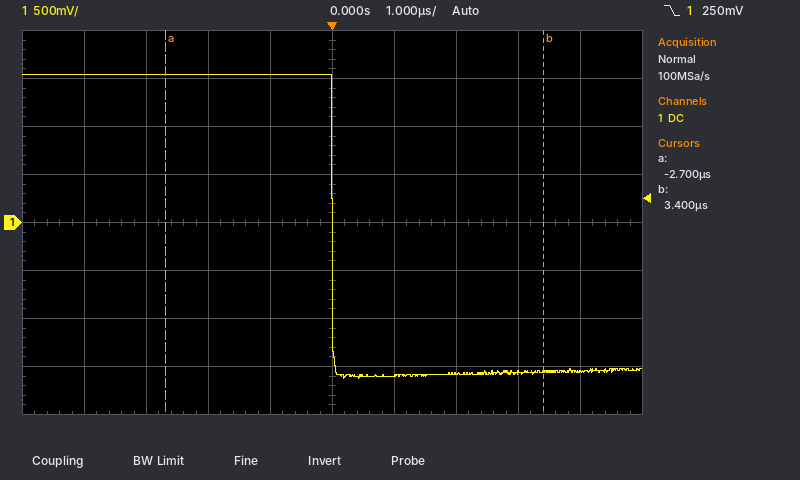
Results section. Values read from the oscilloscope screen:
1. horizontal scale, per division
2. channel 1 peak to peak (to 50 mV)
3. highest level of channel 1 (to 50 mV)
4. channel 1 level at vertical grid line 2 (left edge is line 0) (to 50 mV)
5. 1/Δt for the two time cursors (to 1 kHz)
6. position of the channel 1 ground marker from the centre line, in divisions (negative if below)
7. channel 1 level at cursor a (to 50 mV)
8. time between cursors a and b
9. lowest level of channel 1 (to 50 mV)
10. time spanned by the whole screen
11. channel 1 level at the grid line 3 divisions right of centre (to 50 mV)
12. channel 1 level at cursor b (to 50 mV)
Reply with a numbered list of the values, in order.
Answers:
1. 1 µs
2. 3.15 V
3. 1.55 V
4. 1.55 V
5. 164 kHz
6. 0.0 div
7. 1.55 V
8. 6.1 µs
9. -1.60 V
10. 10 µs
11. -1.55 V
12. -1.55 V
